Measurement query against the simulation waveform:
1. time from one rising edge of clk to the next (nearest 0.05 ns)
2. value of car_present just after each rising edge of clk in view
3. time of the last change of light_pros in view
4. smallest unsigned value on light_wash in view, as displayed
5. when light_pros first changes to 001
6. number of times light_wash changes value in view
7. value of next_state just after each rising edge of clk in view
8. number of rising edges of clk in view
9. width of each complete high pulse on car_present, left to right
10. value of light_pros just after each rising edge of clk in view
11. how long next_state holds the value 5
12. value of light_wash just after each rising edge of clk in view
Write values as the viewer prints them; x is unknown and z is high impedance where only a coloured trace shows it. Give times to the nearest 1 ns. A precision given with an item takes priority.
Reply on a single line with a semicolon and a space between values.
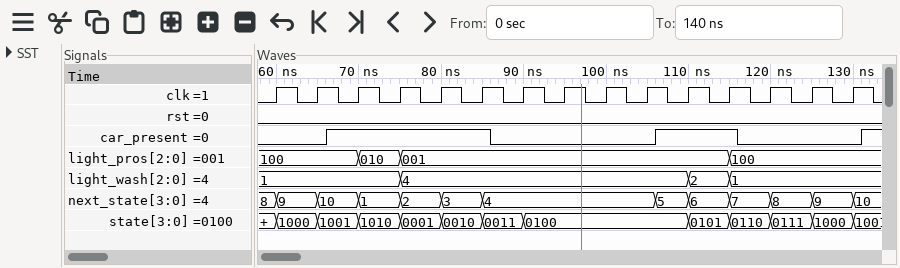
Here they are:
5 ns; 0 0 1 1 1 1 0 0 0 0 1 1 0 0 0; 115 ns; 1; 75 ns; 3; 9, 10, 1, 2, 3, 4, 4, 4, 4, 4, 6, 7, 8, 9, 10; 15; 20 ns, 10 ns; 100, 100, 010, 001, 001, 001, 001, 001, 001, 001, 001, 100, 100, 100, 100; 4 ns; 1, 1, 1, 4, 4, 4, 4, 4, 4, 4, 2, 1, 1, 1, 1
